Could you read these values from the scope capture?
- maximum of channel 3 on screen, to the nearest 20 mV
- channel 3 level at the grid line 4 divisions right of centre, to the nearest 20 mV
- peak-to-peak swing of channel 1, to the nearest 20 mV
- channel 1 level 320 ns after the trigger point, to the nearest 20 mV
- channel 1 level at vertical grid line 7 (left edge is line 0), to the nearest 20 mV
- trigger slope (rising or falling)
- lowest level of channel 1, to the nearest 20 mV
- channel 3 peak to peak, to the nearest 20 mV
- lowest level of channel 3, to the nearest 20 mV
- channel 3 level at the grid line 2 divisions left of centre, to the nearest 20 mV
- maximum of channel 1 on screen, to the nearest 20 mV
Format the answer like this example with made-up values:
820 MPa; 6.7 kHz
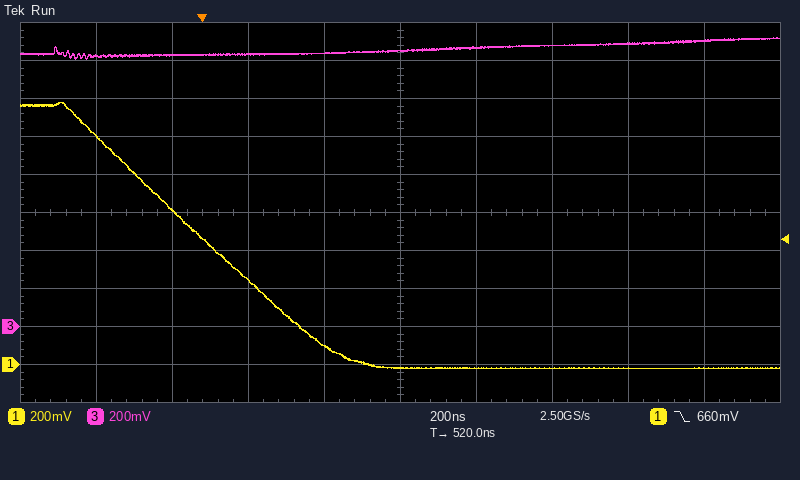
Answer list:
1.52 V; 1.50 V; 1.40 V; 100 mV; -20 mV; falling; -20 mV; 120 mV; 1.40 V; 1.44 V; 1.38 V
